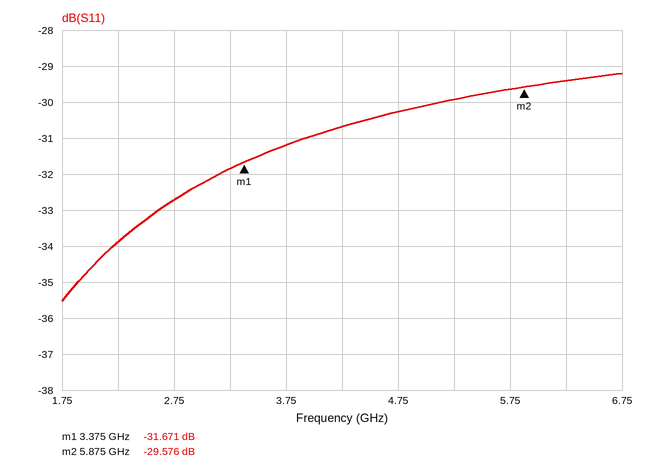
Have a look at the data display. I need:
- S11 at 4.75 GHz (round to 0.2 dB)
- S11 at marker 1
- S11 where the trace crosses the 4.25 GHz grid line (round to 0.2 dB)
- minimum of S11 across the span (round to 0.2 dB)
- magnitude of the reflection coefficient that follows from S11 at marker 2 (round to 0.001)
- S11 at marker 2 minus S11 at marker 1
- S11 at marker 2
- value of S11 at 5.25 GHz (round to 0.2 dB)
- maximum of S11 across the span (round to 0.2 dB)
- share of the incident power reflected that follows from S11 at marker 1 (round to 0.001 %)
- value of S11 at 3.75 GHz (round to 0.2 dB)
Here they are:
-30.2 dB
-31.671 dB
-30.6 dB
-35.6 dB
0.033
2.095 dB
-29.576 dB
-30.0 dB
-29.2 dB
0.068 %
-31.2 dB
